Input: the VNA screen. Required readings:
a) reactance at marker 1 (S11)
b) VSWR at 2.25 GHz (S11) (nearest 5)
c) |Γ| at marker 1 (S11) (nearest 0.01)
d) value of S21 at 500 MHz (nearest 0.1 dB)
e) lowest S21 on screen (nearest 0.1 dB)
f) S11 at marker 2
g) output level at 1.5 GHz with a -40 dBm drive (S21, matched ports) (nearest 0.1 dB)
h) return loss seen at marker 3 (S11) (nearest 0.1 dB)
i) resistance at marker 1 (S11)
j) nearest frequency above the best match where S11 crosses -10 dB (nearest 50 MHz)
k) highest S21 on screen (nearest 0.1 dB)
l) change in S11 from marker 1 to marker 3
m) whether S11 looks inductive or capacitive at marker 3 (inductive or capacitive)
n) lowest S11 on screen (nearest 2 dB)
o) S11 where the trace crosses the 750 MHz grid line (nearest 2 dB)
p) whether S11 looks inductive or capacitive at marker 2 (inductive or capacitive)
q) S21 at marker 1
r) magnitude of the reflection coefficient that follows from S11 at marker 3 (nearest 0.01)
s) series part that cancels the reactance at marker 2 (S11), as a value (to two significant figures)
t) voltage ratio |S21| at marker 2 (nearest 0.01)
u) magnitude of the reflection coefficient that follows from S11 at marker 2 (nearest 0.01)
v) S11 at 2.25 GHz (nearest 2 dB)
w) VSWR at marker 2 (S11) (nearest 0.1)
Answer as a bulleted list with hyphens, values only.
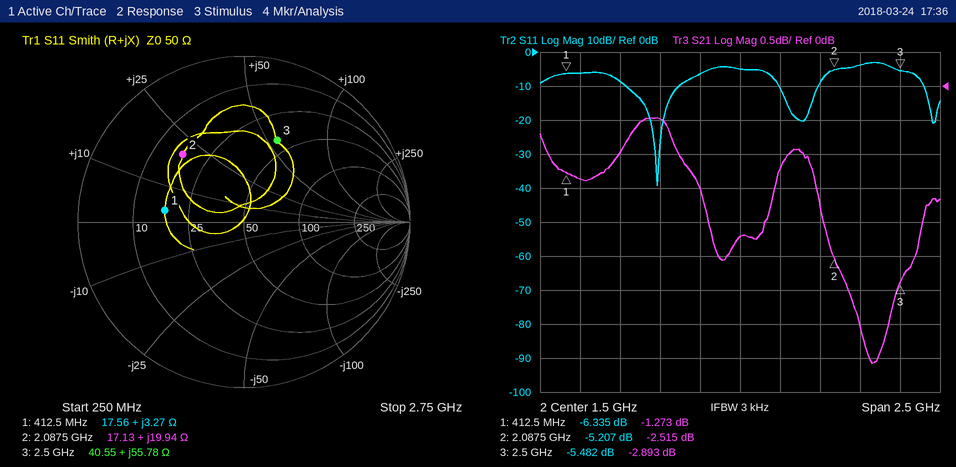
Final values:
- +3.27 Ω
- 5
- 0.48
- -1.4 dB
- -4.1 dB
- -5.207 dB
- -42.2 dBm
- 5.5 dB
- 17.56 Ω
- 1.10 GHz
- -0.5 dB
- 0.853 dB
- inductive
- -40 dB
- -8 dB
- inductive
- -1.273 dB
- 0.53
- 3.8 pF
- 0.75
- 0.55
- -4 dB
- 3.4
